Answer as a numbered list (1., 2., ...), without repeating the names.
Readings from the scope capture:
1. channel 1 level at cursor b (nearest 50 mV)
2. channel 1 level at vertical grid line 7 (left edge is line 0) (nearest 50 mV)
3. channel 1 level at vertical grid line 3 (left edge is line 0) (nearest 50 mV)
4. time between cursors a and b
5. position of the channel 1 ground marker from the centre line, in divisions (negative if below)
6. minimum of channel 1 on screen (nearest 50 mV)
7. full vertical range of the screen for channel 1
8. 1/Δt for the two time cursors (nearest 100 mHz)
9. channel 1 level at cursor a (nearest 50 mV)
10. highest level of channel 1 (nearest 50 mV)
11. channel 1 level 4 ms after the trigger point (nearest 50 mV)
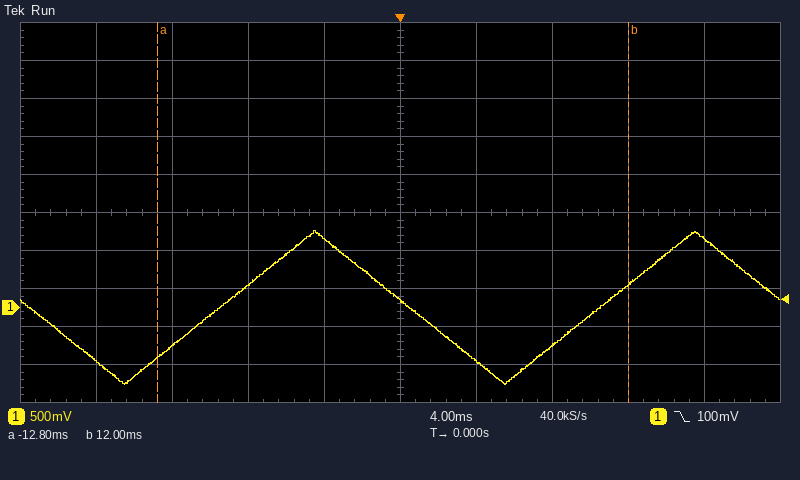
1. 300 mV
2. -500 mV
3. 300 mV
4. 24.8 ms
5. -2.5 div
6. -1.00 V
7. 5 V
8. 40.3 Hz
9. -650 mV
10. 1.00 V
11. -700 mV
